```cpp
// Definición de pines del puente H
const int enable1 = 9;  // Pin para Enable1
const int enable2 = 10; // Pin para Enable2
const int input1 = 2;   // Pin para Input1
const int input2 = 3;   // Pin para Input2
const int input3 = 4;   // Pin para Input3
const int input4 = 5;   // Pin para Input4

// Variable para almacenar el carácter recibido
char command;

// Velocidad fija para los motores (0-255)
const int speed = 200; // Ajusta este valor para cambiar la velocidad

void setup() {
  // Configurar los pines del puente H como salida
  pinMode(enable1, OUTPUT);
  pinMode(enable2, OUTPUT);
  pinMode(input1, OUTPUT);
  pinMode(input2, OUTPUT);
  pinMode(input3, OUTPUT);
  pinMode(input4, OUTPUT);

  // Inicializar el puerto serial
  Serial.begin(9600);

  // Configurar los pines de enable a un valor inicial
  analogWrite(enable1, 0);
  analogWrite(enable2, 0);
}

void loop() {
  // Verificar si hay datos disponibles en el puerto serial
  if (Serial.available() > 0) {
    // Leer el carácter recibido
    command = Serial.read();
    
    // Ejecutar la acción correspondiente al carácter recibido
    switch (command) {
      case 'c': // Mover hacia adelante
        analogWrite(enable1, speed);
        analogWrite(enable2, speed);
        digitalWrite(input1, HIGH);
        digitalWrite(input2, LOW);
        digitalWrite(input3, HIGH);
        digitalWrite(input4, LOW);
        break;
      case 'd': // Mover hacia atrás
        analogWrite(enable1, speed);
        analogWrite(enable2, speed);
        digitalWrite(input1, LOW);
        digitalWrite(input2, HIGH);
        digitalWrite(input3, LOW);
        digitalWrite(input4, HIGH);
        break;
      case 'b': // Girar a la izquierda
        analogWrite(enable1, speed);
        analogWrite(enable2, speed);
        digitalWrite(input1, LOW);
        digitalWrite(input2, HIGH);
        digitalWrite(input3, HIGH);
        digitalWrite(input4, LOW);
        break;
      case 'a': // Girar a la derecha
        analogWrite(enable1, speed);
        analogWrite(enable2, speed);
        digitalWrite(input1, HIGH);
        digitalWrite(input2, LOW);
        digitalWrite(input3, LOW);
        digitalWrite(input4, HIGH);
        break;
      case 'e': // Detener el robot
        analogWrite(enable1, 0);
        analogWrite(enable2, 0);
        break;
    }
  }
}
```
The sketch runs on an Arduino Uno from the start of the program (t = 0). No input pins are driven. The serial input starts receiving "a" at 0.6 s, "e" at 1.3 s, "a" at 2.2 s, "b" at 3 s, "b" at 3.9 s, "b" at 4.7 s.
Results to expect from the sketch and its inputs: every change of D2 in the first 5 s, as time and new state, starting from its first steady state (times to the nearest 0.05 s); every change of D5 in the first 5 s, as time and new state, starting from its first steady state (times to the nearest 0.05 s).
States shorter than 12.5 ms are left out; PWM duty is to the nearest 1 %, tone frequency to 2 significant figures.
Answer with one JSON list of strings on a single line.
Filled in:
["0 s low; 0.6 s high; 3 s low", "0 s low; 0.6 s high; 3 s low"]
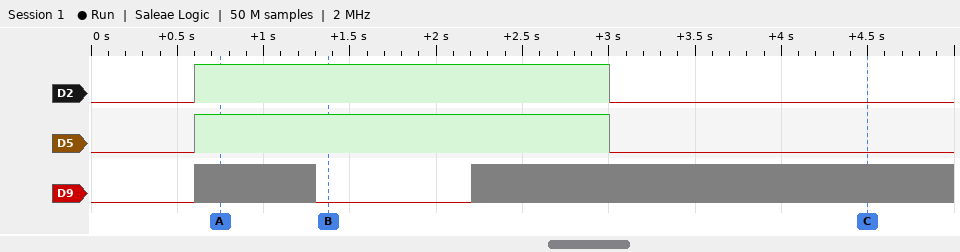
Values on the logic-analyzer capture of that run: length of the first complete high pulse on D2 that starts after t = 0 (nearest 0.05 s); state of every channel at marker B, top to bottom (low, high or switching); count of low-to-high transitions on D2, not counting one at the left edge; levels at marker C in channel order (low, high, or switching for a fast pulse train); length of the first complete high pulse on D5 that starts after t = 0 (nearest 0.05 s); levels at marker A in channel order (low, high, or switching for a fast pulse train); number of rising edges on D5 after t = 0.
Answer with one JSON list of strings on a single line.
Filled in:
["2.40 s", "D2 high, D5 high, D9 low", "1", "D2 low, D5 low, D9 switching", "2.40 s", "D2 high, D5 high, D9 switching", "1"]
